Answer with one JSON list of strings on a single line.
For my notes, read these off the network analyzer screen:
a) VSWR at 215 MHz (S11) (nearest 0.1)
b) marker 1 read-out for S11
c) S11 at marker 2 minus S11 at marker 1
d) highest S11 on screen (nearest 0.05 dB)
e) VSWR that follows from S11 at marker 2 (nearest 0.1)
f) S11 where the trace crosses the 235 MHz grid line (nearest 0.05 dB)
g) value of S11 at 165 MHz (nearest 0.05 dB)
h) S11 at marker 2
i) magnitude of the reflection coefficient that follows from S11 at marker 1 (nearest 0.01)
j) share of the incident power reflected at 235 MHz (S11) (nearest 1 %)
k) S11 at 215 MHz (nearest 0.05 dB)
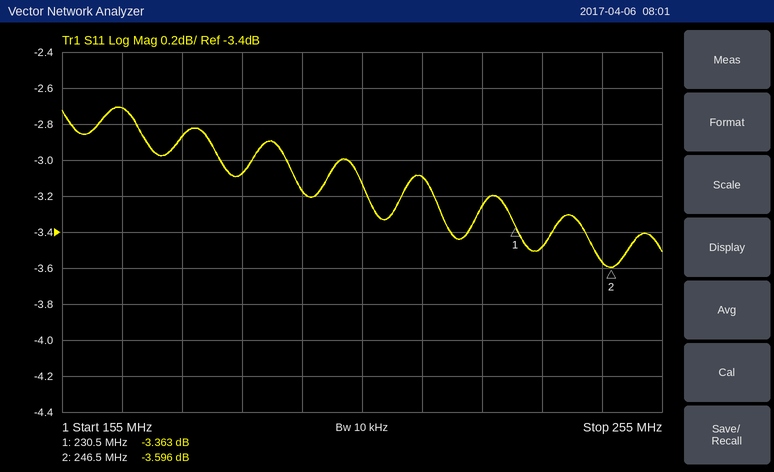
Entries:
["5.7", "-3.363 dB", "-0.233 dB", "-2.70 dB", "4.9", "-3.50 dB", "-2.70 dB", "-3.596 dB", "0.68", "45 %", "-3.10 dB"]
